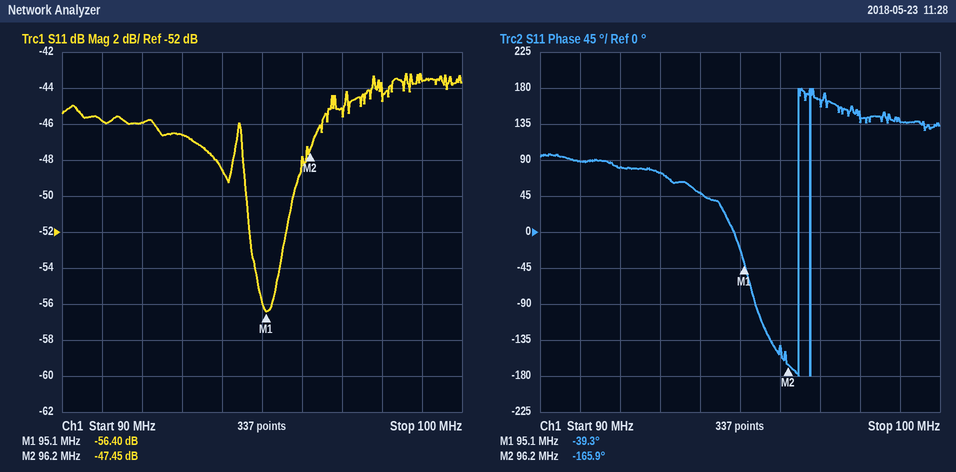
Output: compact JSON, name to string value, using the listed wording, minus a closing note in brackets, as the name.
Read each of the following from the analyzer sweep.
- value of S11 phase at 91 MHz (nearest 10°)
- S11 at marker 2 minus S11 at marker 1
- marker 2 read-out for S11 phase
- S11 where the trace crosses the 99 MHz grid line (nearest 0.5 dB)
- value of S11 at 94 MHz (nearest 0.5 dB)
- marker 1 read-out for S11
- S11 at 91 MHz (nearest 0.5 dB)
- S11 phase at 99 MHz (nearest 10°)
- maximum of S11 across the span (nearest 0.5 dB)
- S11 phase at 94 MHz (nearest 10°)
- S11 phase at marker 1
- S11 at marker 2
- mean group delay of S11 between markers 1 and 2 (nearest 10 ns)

{"value of S11 phase at 91 MHz": "90°", "S11 at marker 2 minus S11 at marker 1": "8.95 dB", "marker 2 read-out for S11 phase": "-165.9°", "S11 where the trace crosses the 99 MHz grid line": "-43.5 dB", "value of S11 at 94 MHz": "-48.5 dB", "marker 1 read-out for S11": "-56.40 dB", "S11 at 91 MHz": "-46.0 dB", "S11 phase at 99 MHz": "140°", "maximum of S11 across the span": "-43.0 dB", "S11 phase at 94 MHz": "50°", "S11 phase at marker 1": "-39.3°", "S11 at marker 2": "-47.45 dB", "mean group delay of S11 between markers 1 and 2": "320 ns"}
